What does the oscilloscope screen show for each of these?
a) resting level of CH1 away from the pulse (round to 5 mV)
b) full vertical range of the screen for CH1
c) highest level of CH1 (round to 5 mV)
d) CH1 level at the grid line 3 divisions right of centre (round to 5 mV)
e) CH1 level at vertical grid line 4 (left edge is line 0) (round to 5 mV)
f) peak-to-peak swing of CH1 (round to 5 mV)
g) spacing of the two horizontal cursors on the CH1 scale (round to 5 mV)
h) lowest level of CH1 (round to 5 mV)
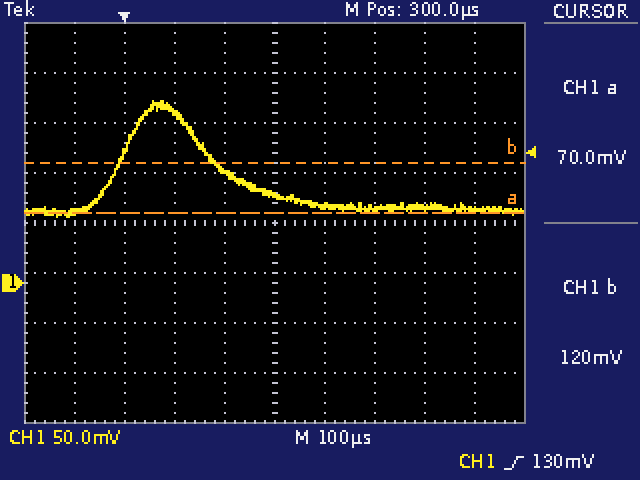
75 mV
400 mV
180 mV
75 mV
110 mV
115 mV
50 mV
65 mV
